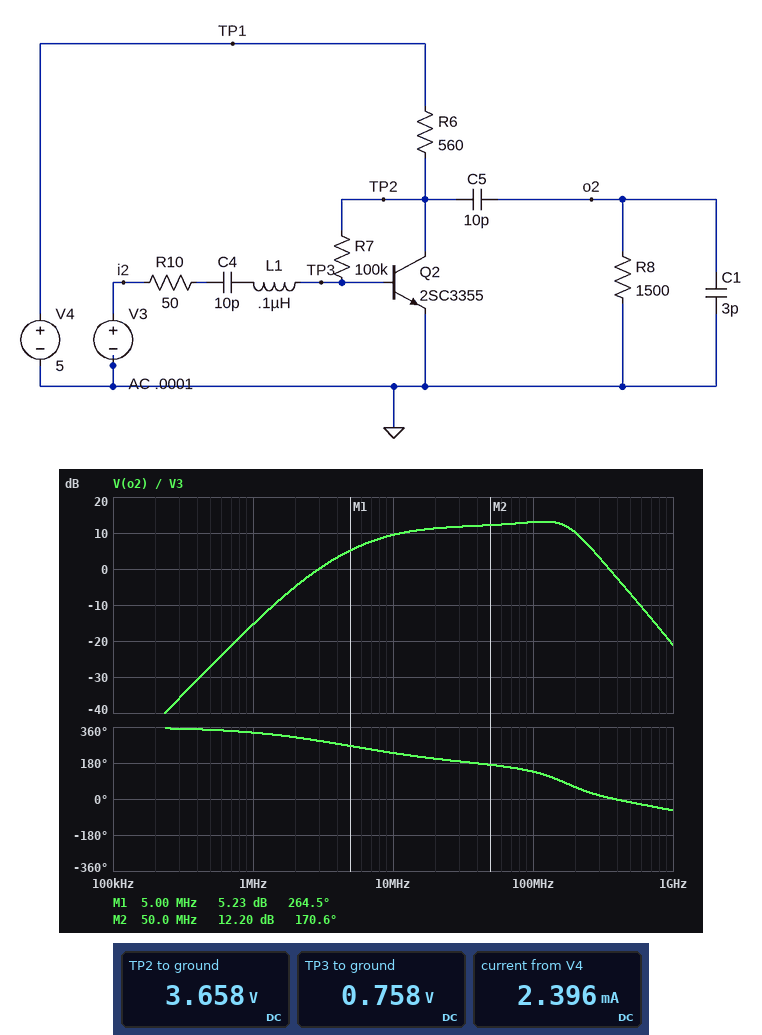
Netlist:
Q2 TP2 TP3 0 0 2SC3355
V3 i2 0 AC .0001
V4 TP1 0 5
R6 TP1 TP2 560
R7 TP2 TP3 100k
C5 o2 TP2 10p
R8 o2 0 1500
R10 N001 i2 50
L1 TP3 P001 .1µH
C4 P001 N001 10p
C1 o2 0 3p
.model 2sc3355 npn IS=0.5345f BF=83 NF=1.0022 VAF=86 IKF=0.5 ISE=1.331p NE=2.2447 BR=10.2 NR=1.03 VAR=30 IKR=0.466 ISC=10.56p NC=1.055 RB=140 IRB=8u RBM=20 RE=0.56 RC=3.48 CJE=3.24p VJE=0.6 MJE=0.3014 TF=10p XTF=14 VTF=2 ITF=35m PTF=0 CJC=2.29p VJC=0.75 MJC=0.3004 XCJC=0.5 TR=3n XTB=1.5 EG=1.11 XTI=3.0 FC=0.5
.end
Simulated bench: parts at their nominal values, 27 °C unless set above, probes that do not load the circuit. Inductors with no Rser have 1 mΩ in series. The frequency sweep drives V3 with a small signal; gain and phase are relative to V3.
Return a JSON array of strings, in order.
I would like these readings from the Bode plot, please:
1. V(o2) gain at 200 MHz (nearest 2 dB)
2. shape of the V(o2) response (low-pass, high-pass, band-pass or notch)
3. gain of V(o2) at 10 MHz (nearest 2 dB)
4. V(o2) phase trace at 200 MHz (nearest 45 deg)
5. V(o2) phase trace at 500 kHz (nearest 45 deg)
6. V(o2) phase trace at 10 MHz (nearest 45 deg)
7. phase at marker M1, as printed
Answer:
["10 dB", "band-pass", "10 dB", "45 deg", "360 deg", "225 deg", "264.5 deg"]
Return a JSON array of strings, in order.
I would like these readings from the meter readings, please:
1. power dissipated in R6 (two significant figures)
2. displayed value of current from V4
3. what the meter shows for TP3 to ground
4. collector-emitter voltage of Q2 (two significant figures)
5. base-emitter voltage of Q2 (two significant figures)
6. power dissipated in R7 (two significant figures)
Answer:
["3.2 mW", "2.396 mA", "0.758 V", "3.7 V", "760 mV", "84 µW"]
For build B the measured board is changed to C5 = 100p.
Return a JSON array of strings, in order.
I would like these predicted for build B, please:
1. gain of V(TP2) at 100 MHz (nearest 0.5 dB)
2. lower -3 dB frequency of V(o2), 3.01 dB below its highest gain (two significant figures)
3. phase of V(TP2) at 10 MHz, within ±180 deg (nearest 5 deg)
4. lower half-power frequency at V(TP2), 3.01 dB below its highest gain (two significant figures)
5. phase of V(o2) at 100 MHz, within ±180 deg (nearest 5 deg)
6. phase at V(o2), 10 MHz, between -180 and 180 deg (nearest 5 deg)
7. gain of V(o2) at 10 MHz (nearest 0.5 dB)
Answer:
["15.0 dB", "4.6 MHz", "-165 deg", "4.3 MHz", "130 deg", "-160 deg", "13.5 dB"]
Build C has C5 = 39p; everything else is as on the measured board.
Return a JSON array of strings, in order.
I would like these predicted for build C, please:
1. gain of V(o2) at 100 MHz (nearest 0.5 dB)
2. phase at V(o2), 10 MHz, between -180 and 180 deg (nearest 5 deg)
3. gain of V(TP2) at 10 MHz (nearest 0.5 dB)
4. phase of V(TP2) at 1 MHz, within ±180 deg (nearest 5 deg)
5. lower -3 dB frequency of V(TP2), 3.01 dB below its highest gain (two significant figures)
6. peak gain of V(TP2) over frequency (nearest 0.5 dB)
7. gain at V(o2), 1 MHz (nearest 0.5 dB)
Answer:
["14.5 dB", "-155 deg", "13.5 dB", "-115 deg", "4.2 MHz", "15.0 dB", "-4.5 dB"]
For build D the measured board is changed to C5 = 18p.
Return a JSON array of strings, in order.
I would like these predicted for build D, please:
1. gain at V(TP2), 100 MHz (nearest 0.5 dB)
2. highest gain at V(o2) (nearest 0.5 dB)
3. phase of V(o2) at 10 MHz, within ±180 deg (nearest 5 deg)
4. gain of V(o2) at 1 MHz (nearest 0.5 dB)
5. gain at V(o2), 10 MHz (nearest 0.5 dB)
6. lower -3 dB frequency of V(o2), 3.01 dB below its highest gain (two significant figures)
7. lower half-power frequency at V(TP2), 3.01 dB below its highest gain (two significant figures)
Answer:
["15.0 dB", "14.0 dB", "-140 deg", "-10.5 dB", "11.5 dB", "8.4 MHz", "3.9 MHz"]
